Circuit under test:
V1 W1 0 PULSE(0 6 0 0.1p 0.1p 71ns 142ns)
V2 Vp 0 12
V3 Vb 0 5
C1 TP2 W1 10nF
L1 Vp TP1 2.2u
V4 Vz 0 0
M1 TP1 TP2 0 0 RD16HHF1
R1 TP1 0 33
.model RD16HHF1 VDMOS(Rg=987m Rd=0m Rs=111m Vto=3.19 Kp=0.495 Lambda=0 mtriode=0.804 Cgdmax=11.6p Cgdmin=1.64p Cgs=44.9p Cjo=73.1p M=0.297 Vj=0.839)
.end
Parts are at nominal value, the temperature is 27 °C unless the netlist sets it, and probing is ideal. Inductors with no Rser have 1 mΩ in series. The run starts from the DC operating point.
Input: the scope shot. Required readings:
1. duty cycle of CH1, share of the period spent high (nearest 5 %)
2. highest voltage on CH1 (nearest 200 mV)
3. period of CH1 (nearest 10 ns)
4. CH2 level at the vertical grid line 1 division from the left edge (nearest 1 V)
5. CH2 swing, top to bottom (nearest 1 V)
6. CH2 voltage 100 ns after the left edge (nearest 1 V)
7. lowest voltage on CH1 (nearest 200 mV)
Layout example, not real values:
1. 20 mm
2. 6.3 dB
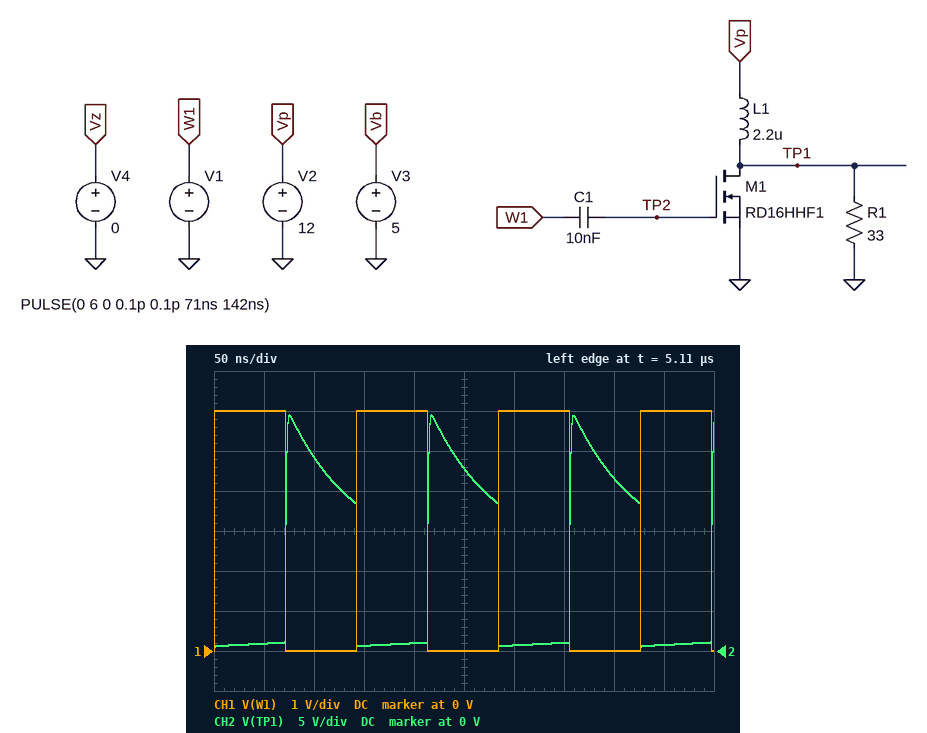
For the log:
1. 50 %
2. 6.0 V
3. 140 ns
4. 1 V
5. 29 V
6. 24 V
7. 0 V
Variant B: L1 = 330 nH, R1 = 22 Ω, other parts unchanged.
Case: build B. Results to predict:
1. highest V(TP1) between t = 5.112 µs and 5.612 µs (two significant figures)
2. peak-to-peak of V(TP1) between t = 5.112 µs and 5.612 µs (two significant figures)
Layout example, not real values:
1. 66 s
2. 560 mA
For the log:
1. 45 V
2. 44 V
